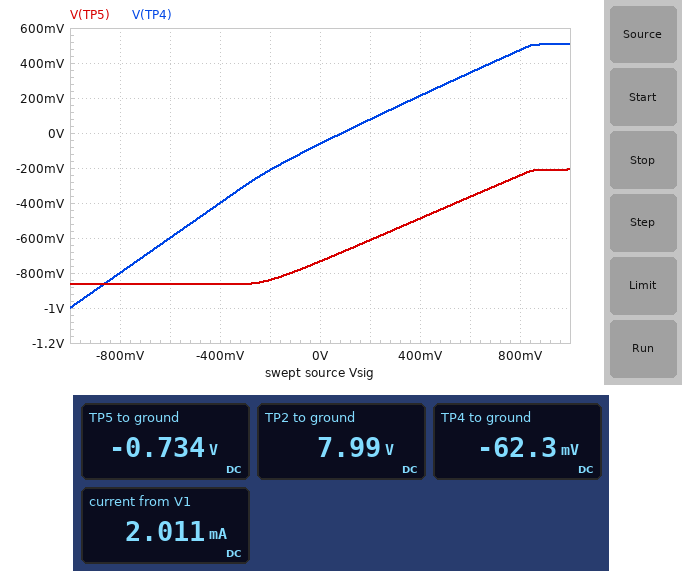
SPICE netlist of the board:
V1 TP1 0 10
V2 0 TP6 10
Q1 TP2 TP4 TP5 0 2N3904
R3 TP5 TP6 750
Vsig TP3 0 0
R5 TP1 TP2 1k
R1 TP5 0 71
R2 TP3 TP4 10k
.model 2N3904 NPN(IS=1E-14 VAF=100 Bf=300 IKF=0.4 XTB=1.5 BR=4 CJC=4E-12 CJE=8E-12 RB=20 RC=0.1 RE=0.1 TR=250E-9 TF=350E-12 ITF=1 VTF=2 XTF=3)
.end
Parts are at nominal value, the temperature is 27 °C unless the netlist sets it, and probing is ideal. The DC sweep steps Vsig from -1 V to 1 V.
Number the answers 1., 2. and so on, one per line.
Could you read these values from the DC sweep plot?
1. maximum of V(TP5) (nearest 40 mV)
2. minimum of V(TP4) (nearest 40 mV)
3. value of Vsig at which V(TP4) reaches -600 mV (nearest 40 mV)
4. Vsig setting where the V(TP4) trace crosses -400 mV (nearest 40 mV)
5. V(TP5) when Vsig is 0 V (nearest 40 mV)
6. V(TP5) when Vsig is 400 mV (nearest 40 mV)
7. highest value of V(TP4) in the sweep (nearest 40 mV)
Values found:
1. -200 mV
2. -1.00 V
3. -600 mV
4. -400 mV
5. -720 mV
6. -480 mV
7. 520 mV
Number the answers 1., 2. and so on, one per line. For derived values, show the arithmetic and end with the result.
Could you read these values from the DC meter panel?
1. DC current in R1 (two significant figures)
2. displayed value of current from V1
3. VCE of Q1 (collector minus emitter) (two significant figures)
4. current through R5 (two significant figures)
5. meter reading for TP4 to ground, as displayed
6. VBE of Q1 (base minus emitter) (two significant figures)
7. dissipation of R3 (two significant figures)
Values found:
1. (0 V - (-734 mV)) / 71 Ω = 10 mA
2. 2.011 mA
3. 7.99 V - (-734 mV) = 8.7 V
4. (10 V - 7.99 V) / 1 kΩ = 2.0 mA
5. -62.3 mV
6. -62.3 mV - (-734 mV) = 670 mV
7. (-734 mV - (-10 V))^2 / 750 Ω = 110 mW
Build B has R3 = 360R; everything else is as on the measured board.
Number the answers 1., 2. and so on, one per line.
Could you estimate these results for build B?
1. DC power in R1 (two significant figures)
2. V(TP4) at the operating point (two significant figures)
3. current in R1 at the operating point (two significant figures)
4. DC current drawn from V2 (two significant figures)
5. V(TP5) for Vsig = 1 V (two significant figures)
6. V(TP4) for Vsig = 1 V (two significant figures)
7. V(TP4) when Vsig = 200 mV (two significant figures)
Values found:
1. 16 mW
2. -340 mV
3. 15 mA
4. 25 mA
5. -990 mV
6. -270 mV
7. -280 mV
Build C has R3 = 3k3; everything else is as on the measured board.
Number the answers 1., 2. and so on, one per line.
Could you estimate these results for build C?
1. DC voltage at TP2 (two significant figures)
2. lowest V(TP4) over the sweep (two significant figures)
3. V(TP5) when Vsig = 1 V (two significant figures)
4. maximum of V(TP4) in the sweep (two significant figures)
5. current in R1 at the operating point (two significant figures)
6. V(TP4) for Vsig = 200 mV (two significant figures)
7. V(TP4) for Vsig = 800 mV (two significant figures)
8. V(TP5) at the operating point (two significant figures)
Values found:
1. 10 V
2. -1.0 V
3. 140 mV
4. 840 mV
5. 3.0 mA
6. 200 mV
7. 700 mV
8. -210 mV
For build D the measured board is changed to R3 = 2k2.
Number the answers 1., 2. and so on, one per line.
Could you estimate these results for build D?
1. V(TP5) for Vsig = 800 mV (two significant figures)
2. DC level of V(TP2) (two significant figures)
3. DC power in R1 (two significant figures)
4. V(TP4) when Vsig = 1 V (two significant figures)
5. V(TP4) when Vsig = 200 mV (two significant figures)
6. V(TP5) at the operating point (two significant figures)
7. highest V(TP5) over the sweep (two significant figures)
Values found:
1. -25 mV
2. 10 V
3. 1.4 mW
4. 800 mV
5. 200 mV
6. -310 mV
7. 100 mV
